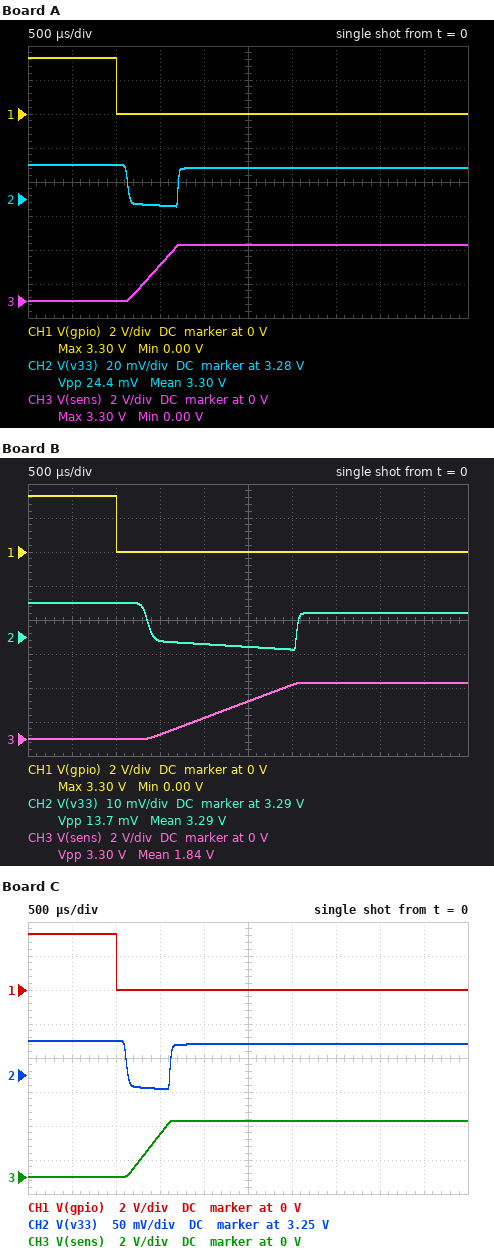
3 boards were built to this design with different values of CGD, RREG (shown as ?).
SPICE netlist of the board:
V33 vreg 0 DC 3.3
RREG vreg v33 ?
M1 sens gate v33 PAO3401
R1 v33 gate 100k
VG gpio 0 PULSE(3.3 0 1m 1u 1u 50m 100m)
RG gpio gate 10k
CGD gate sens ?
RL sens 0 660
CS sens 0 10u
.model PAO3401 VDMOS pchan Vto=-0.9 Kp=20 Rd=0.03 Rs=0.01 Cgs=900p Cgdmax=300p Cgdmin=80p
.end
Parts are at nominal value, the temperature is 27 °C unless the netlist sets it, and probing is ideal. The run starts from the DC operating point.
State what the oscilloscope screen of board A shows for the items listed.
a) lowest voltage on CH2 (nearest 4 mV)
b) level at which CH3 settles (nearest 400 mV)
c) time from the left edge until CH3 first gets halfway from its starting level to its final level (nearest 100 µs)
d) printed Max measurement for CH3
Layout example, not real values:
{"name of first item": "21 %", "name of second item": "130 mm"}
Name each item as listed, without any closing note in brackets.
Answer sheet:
{"lowest voltage on CH2": "3.276 V", "level at which CH3 settles": "3.2 V", "time from the left edge until CH3 first gets halfway from its starting level to its final level": "1.4 ms", "printed Max measurement for CH3": "3.30 V"}
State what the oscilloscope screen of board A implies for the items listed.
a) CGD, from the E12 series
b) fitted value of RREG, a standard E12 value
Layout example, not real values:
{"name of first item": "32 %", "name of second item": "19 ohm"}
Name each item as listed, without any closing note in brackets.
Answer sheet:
{"CGD, from the E12 series": "39 nF", "fitted value of RREG, a standard E12 value": "0.39 Ω"}
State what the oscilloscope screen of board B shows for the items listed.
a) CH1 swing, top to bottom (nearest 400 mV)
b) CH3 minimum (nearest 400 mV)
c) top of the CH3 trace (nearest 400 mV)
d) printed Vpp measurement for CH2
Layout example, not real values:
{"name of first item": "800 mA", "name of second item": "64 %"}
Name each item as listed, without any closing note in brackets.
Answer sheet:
{"CH1 swing, top to bottom": "3.2 V", "CH3 minimum": "0 V", "top of the CH3 trace": "3.2 V", "printed Vpp measurement for CH2": "13.7 mV"}
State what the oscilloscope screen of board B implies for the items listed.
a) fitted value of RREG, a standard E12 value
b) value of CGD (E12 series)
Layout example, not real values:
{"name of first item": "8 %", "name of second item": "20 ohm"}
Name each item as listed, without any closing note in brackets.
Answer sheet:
{"fitted value of RREG, a standard E12 value": "0.56 Ω", "value of CGD": "120 nF"}
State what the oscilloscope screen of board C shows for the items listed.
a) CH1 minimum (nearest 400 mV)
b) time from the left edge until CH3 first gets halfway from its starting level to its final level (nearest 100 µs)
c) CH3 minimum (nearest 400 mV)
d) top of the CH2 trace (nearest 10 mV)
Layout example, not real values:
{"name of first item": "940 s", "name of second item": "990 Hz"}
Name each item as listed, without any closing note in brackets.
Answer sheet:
{"CH1 minimum": "0 V", "time from the left edge until CH3 first gets halfway from its starting level to its final level": "1.4 ms", "CH3 minimum": "0 V", "top of the CH2 trace": "3.30 V"}
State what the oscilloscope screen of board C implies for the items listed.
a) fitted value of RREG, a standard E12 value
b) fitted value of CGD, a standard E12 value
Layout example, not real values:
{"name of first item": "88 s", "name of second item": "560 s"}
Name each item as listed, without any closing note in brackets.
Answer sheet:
{"fitted value of RREG, a standard E12 value": "1 Ω", "fitted value of CGD, a standard E12 value": "33 nF"}
